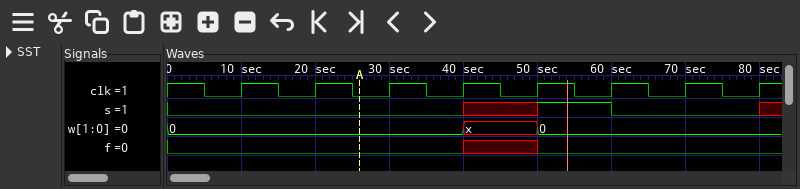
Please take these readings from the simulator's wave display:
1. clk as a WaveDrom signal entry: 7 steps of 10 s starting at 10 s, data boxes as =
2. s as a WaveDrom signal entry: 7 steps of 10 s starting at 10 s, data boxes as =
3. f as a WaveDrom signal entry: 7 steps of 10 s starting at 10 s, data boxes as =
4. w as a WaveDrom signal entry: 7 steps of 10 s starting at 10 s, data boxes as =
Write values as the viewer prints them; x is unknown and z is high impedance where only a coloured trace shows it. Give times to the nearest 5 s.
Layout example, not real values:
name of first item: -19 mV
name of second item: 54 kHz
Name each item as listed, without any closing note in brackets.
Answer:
clk as a WaveDrom signal entry: 7 steps of 10 s starting at 10 s, data boxes as =: {name: 'clk', wave: 'p......'}
s as a WaveDrom signal entry: 7 steps of 10 s starting at 10 s, data boxes as =: {name: 's', wave: '0..x10.'}
f as a WaveDrom signal entry: 7 steps of 10 s starting at 10 s, data boxes as =: {name: 'f', wave: '0..x0..'}
w as a WaveDrom signal entry: 7 steps of 10 s starting at 10 s, data boxes as =: {name: 'w', wave: '=..x=..', data: '0 0'}
